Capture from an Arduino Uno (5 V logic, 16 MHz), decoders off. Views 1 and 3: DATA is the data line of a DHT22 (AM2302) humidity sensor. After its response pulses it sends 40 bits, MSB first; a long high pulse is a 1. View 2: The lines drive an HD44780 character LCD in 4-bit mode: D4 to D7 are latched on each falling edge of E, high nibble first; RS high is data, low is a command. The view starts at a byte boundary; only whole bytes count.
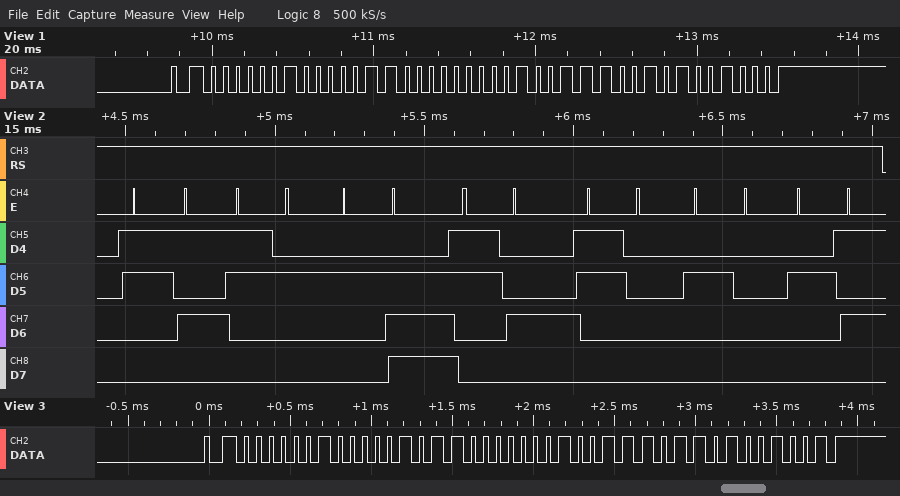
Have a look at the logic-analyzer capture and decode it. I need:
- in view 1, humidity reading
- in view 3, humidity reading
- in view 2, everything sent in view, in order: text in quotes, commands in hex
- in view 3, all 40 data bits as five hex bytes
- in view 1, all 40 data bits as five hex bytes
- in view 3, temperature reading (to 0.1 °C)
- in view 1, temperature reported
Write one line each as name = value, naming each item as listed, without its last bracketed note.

in view 1, humidity reading = 52.4 %
in view 3, humidity reading = 52.3 %
in view 2, everything sent in view, in order: text in quotes, commands in hex = "52.40 %"
in view 3, all 40 data bits as five hex bytes = 02 0B 01 3B 49
in view 1, all 40 data bits as five hex bytes = 02 0C 01 39 48
in view 3, temperature reading = 31.5 °C
in view 1, temperature reported = 31.3 °C
